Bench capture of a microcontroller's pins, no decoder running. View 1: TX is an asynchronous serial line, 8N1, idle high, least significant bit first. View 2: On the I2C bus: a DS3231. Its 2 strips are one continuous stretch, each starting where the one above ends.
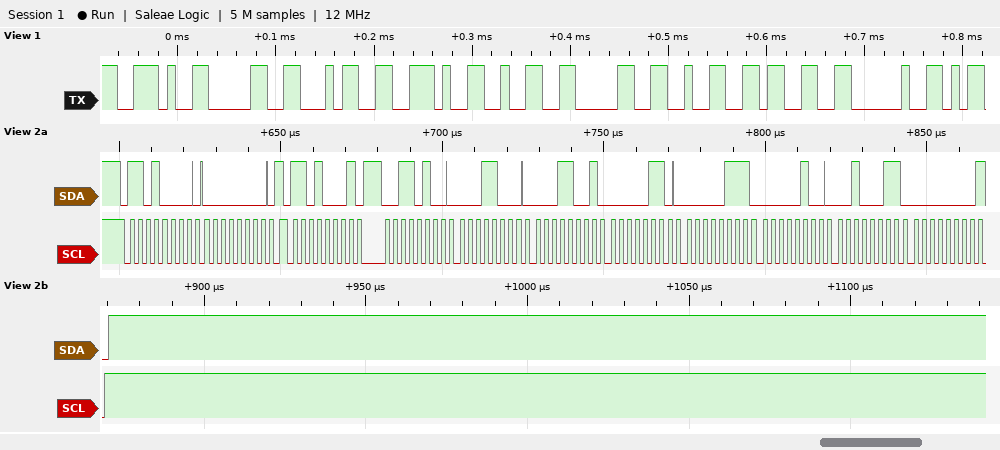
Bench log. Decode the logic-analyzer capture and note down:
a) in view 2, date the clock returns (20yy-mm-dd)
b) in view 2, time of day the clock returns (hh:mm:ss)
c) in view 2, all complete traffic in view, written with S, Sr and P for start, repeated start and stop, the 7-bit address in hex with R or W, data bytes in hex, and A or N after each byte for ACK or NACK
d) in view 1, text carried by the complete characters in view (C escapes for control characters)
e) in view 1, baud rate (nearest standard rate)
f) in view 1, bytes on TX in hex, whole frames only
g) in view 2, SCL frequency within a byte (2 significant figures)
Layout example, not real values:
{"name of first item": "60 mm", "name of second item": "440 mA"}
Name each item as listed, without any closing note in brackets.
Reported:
{"in view 2, date the clock returns": "2023-04-07", "in view 2, time of day the clock returns": "19:18:34", "in view 2, all complete traffic in view, written with S, Sr and P for start, repeated start and stop, the 7-bit address in hex with R or W, data bytes in hex, and A or N after each byte for ACK or NACK": "S 68W A 00 A Sr 68R A 34 A 18 A 19 A 06 A 07 A 04 A 23 A 00 N P", "in view 1, text carried by the complete characters in view": "\".04.2023 \"", "in view 1, baud rate": "115200 baud", "in view 1, bytes on TX in hex, whole frames only": "0x2E 0x30 0x34 0x2E 0x32 0x30 0x32 0x33 0x20", "in view 2, SCL frequency within a byte": "400 kHz"}
